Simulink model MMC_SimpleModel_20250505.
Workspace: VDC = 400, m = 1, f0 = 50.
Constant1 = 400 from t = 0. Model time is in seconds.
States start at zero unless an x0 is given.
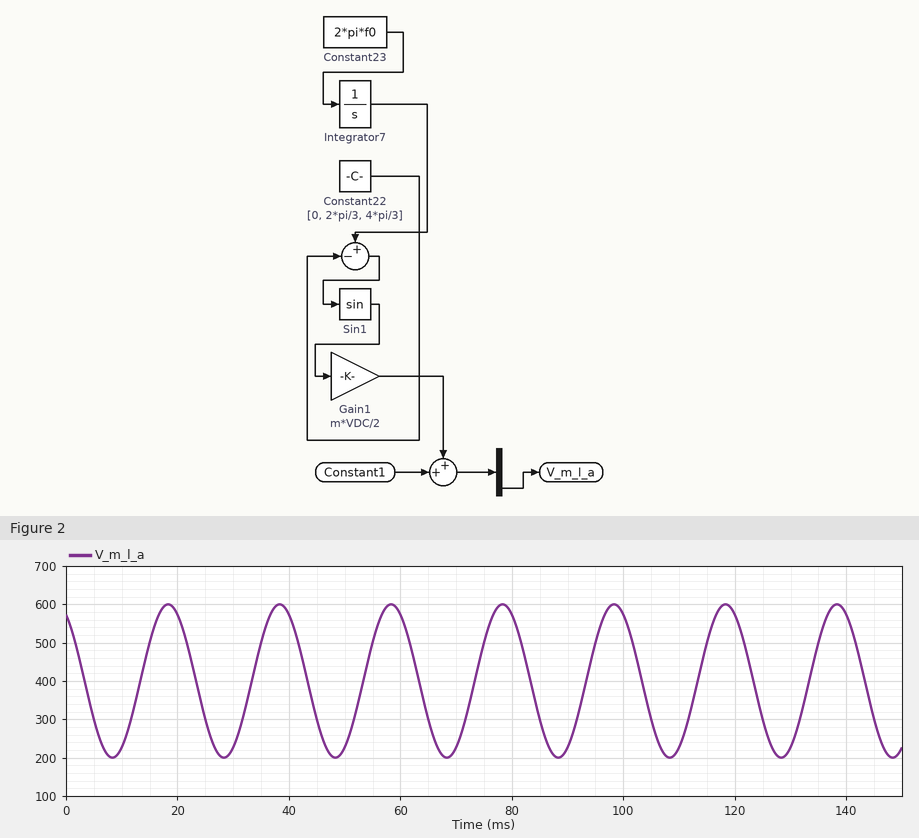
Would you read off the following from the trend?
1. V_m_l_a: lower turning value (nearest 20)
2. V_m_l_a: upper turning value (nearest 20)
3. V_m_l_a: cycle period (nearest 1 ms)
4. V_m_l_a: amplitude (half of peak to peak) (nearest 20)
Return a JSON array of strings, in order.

["200", "600", "20 ms", "200"]
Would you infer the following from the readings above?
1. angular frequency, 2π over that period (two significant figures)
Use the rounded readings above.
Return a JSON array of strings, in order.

["0.31 rad/ms"]
